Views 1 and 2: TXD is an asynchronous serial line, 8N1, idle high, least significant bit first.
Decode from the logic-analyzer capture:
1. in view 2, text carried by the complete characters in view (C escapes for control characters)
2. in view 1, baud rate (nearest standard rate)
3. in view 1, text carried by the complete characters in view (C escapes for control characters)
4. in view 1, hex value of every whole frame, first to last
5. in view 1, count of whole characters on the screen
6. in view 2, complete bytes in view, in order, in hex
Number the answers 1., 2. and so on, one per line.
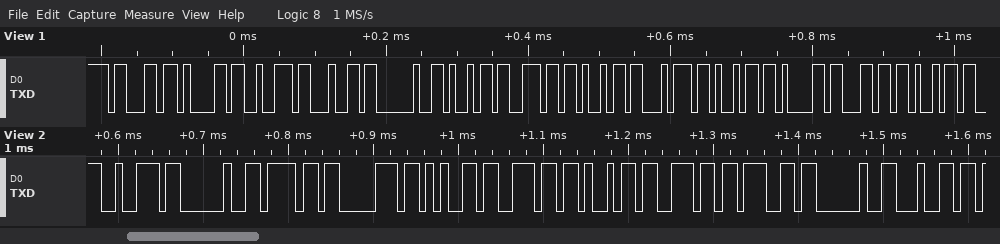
1. "r opening d"
2. 115200 baud
3. "card initiali"
4. 63 61 72 64 20 69 6E 69 74 69 61 6C 69
5. 13
6. 72 20 6F 70 65 6E 69 6E 67 20 64
